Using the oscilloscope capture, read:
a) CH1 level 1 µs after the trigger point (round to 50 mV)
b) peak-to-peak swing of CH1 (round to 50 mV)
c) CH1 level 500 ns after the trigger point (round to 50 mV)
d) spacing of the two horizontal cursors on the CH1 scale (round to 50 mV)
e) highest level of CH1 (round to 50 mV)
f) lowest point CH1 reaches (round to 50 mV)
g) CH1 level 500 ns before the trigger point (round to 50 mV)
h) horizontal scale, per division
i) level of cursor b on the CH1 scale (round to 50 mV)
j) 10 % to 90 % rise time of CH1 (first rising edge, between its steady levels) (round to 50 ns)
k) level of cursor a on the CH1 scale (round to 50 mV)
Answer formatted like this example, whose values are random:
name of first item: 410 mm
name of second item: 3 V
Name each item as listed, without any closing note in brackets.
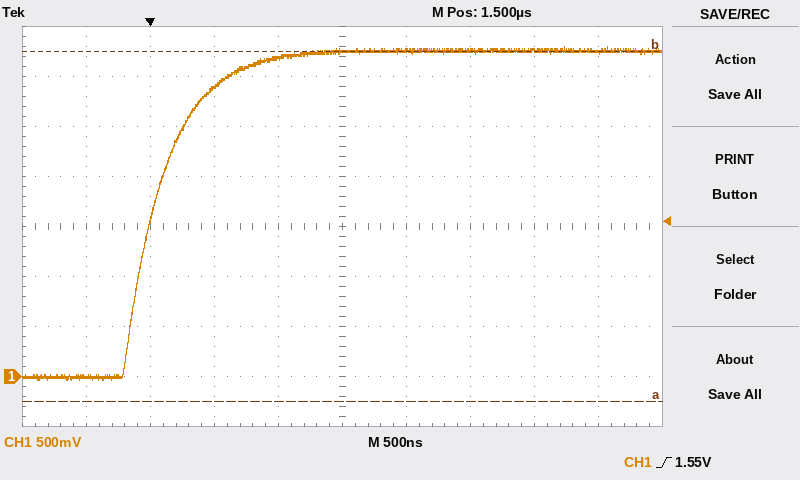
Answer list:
CH1 level 1 µs after the trigger point: 3.20 V
peak-to-peak swing of CH1: 3.35 V
CH1 level 500 ns after the trigger point: 2.90 V
spacing of the two horizontal cursors on the CH1 scale: 3.50 V
highest level of CH1: 3.30 V
lowest point CH1 reaches: -50 mV
CH1 level 500 ns before the trigger point: 0 mV
horizontal scale, per division: 500 ns
level of cursor b on the CH1 scale: 3.25 V
10 % to 90 % rise time of CH1 (first rising edge, between its steady levels): 700 ns
level of cursor a on the CH1 scale: -250 mV
